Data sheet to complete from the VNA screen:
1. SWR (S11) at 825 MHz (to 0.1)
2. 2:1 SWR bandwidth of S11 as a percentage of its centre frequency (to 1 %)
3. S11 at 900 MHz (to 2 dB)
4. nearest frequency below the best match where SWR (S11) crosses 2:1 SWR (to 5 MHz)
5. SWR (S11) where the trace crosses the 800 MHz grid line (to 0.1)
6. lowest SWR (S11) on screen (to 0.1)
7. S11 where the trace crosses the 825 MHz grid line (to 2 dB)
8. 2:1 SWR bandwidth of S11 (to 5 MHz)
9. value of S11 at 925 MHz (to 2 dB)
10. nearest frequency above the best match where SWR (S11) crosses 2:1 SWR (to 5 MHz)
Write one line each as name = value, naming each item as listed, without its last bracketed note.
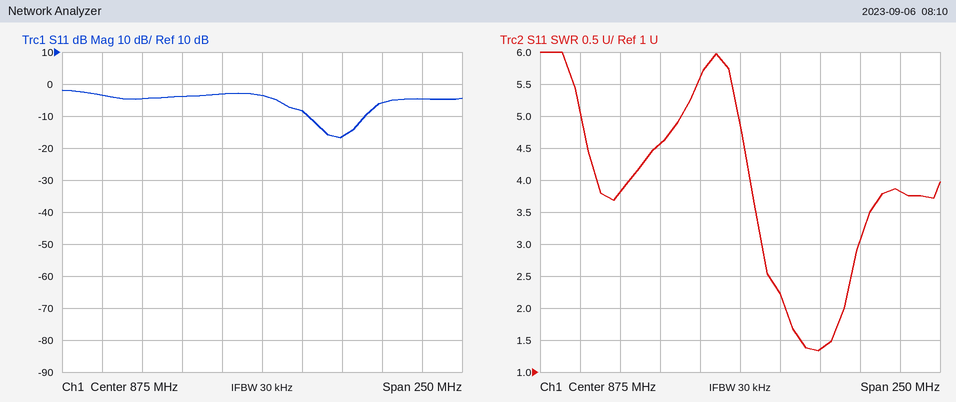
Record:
SWR (S11) at 825 MHz = 4.6
2:1 SWR bandwidth of S11 as a percentage of its centre frequency = 4 %
S11 at 900 MHz = -8 dB
nearest frequency below the best match where SWR (S11) crosses 2:1 SWR = 905 MHz
SWR (S11) where the trace crosses the 800 MHz grid line = 3.8
lowest SWR (S11) on screen = 1.3
S11 where the trace crosses the 825 MHz grid line = -4 dB
2:1 SWR bandwidth of S11 = 35 MHz
value of S11 at 925 MHz = -16 dB
nearest frequency above the best match where SWR (S11) crosses 2:1 SWR = 940 MHz
